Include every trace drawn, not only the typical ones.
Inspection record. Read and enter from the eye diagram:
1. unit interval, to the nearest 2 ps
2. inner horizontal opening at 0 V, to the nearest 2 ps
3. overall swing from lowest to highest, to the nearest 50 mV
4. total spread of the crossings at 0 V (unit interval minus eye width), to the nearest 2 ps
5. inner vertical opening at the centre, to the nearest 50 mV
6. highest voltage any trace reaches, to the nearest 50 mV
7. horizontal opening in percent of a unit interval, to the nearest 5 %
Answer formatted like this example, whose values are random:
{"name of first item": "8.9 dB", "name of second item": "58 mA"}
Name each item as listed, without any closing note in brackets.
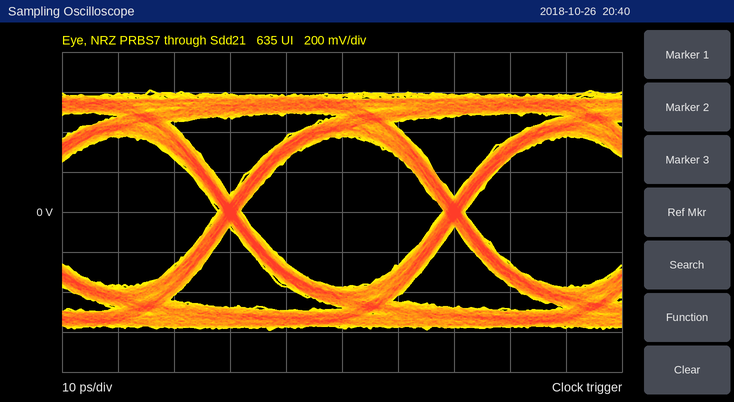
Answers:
{"unit interval, to the nearest 2 ps": "40 ps", "inner horizontal opening at 0 V, to the nearest 2 ps": "36 ps", "overall swing from lowest to highest, to the nearest 50 mV": "1.20 V", "total spread of the crossings at 0 V (unit interval minus eye width), to the nearest 2 ps": "4 ps", "inner vertical opening at the centre, to the nearest 50 mV": "750 mV", "highest voltage any trace reaches, to the nearest 50 mV": "600 mV", "horizontal opening in percent of a unit interval, to the nearest 5 %": "90 %"}
